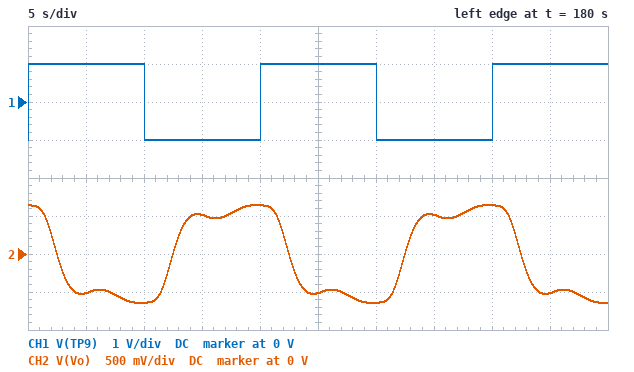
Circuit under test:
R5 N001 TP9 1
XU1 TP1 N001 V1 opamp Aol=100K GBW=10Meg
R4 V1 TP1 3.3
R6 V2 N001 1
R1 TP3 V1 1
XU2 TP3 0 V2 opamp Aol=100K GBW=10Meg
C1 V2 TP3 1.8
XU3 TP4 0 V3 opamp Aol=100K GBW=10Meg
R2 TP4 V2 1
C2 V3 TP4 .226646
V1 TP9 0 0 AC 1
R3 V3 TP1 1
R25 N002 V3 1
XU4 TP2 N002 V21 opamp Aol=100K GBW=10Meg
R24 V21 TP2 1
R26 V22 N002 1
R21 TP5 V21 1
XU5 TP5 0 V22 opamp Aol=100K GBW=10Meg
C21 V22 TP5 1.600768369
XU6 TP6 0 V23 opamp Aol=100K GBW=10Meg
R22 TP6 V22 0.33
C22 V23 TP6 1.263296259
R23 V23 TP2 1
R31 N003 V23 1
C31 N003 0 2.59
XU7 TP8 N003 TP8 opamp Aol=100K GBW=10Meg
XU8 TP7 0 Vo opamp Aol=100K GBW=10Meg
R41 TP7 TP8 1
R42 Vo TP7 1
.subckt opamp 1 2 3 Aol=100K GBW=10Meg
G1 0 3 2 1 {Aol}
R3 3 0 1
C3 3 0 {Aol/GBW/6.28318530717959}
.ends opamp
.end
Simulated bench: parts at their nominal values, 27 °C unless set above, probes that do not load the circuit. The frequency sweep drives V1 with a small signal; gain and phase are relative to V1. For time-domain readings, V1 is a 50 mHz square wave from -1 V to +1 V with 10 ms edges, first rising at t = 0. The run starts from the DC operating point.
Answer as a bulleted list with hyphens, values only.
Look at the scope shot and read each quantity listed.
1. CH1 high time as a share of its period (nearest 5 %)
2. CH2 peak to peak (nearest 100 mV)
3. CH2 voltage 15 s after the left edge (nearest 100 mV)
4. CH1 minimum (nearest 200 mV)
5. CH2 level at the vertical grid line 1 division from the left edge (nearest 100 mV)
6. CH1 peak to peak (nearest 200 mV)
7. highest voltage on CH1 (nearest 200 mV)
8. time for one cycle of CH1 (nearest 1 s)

- 50 %
- 1.3 V
- 500 mV
- -1.0 V
- -500 mV
- 2.0 V
- 1.0 V
- 20 s
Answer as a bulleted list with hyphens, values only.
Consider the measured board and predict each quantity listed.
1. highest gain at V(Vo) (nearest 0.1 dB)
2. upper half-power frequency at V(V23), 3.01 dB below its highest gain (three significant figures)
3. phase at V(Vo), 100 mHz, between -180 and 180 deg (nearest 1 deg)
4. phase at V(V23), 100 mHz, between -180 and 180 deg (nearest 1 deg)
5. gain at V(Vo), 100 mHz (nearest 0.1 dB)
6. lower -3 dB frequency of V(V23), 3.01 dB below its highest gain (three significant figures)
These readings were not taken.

- -3.7 dB
- 237 mHz
- 96 deg
- -25 deg
- -6.8 dB
- 132 mHz
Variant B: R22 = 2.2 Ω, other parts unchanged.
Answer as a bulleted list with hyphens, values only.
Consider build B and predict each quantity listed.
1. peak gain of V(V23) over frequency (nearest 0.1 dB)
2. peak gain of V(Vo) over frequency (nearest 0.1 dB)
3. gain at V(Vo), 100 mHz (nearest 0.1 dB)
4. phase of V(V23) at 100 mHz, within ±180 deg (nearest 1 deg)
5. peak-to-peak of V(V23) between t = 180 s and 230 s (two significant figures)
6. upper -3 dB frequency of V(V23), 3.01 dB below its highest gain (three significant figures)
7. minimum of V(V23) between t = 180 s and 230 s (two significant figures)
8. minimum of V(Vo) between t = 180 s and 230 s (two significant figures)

- -3.6 dB
- -3.7 dB
- -14.5 dB
- -119 deg
- 1.5 V
- 81.8 mHz
- -740 mV
- -630 mV
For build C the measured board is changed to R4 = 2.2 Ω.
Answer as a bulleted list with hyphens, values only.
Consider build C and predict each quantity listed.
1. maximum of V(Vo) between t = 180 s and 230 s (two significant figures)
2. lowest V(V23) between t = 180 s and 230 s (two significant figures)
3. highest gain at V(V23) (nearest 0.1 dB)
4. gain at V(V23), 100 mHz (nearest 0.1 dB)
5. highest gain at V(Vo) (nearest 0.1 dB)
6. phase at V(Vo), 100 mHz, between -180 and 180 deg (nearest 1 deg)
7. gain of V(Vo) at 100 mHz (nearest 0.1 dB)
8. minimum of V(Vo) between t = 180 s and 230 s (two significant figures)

- 720 mV
- -1.7 V
- 5.6 dB
- 0 dB
- -2.8 dB
- 96 deg
- -5.6 dB
- -720 mV
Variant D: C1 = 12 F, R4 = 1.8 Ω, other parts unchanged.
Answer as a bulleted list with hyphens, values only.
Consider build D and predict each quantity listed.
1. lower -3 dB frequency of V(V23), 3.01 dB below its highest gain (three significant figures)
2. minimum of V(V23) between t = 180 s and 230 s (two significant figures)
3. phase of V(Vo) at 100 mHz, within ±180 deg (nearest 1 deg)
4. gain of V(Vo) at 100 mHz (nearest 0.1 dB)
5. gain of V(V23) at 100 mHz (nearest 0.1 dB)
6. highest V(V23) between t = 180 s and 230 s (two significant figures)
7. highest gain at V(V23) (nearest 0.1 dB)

- 120 mHz
- -2.8 V
- 87 deg
- 1.9 dB
- 7.5 dB
- 2.8 V
- 18.4 dB
